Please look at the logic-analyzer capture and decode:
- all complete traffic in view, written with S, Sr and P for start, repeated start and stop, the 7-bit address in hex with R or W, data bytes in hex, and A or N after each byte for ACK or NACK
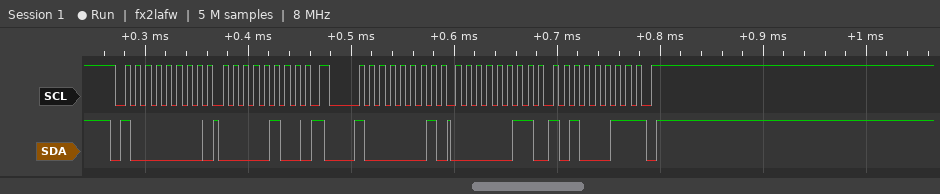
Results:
S 40W A 04 A Sr 40R A 03 A A3 N P
